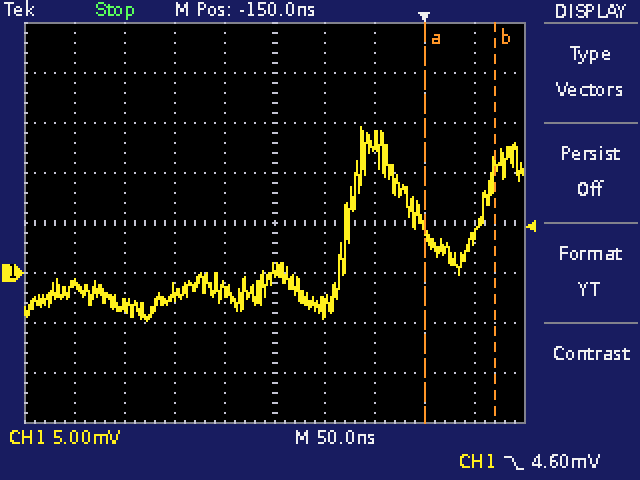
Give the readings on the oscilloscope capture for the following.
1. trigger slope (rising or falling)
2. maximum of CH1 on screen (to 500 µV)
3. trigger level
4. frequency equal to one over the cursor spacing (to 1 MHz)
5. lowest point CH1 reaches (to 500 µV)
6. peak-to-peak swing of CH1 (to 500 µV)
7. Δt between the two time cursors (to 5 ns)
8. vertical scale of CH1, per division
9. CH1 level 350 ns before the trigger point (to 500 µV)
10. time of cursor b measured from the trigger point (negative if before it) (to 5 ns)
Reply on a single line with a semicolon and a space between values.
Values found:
falling; 14.5 mV; 4.60 mV; 14 MHz; -5.0 mV; 19.5 mV; 70 ns; 5 mV; -1.0 mV; +70 ns
